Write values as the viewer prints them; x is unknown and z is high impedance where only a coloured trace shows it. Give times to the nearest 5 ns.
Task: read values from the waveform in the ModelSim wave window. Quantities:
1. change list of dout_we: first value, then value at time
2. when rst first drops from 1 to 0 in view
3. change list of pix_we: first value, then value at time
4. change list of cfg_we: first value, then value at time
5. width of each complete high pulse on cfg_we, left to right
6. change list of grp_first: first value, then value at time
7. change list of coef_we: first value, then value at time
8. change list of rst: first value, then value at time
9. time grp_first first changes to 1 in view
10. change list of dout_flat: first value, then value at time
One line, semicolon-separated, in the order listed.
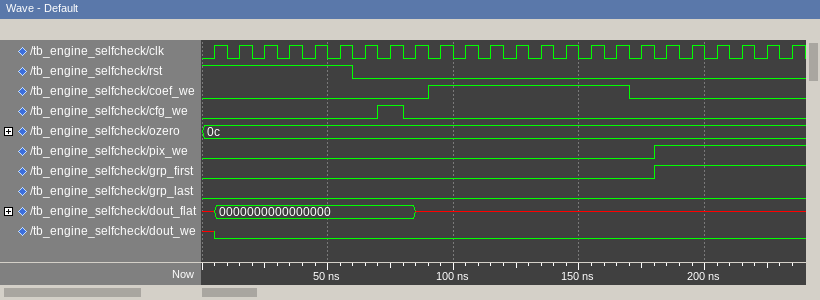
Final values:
x, 0 at 5 ns; 60 ns; 0, 1 at 180 ns; 0, 1 at 70 ns, 0 at 80 ns; 10 ns; 0, 1 at 180 ns; 0, 1 at 90 ns, 0 at 170 ns; 1, 0 at 60 ns; 180 ns; x, 0000000000000000 at 5 ns, x at 85 ns
